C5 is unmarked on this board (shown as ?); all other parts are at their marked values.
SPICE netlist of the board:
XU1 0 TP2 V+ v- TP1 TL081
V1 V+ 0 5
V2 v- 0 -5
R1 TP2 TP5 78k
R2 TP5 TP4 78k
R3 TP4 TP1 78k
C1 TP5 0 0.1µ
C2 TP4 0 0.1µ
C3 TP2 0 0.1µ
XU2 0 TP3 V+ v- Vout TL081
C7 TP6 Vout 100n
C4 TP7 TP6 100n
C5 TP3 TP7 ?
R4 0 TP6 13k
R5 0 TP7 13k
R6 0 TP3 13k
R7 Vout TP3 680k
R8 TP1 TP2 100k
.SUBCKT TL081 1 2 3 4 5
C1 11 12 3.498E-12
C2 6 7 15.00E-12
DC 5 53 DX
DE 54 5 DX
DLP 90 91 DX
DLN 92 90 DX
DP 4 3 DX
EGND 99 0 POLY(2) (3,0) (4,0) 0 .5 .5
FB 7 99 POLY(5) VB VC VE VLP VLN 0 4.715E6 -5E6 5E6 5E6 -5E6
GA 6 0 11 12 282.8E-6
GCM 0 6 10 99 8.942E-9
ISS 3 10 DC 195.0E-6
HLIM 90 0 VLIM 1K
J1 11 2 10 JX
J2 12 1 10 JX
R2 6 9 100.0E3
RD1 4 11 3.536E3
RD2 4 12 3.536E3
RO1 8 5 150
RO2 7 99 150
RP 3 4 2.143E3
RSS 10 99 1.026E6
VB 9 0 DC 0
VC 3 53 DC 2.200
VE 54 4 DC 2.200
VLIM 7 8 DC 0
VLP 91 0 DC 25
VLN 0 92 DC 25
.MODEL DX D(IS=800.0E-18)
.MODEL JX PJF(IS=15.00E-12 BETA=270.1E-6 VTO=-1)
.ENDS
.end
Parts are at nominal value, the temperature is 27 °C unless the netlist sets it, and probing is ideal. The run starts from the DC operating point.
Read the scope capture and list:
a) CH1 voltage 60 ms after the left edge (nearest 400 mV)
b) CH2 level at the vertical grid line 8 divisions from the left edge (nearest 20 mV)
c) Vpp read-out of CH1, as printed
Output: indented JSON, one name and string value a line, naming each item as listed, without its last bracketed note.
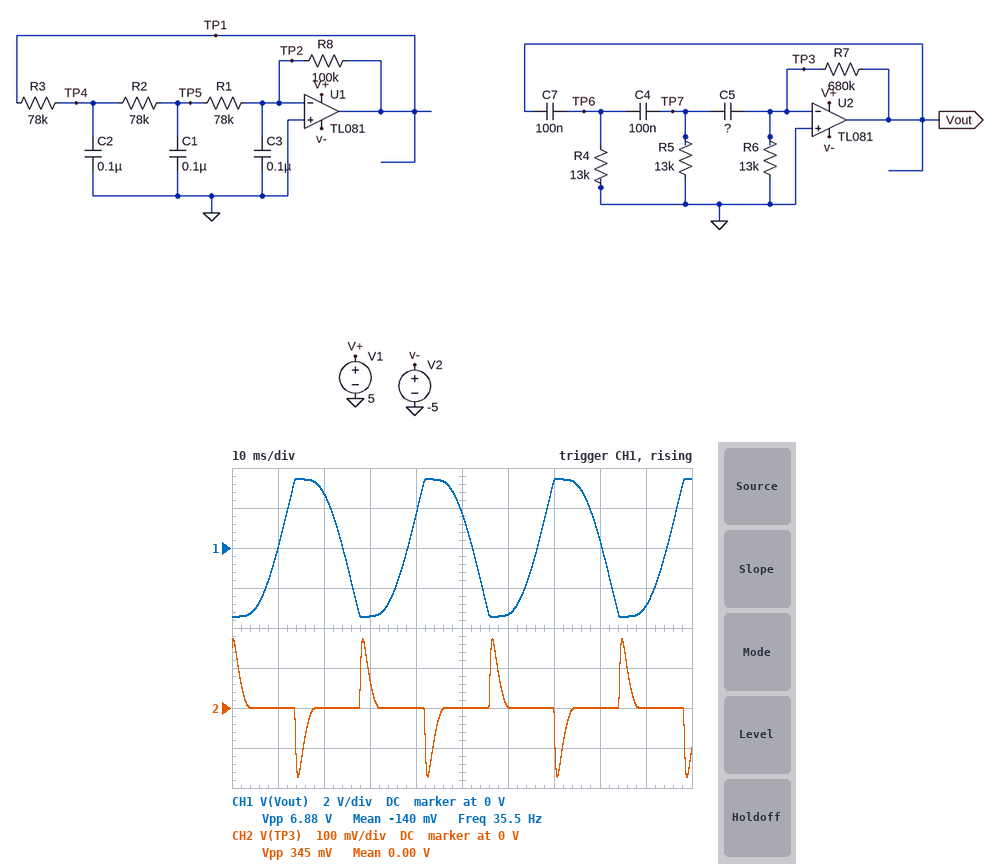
{
  "CH1 voltage 60 ms after the left edge": "-3.2 V",
  "CH2 level at the vertical grid line 8 divisions from the left edge": "0 V",
  "Vpp read-out of CH1, as printed": "6.88 V"
}
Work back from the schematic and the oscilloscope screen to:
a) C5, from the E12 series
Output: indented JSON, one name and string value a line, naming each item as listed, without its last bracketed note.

{
  "C5, from the E12 series": "220 nF"
}
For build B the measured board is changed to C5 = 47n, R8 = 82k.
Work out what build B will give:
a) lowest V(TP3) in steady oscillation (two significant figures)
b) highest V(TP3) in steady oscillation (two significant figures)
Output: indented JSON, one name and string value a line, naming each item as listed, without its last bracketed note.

{
  "lowest V(TP3) in steady oscillation": "-210 mV",
  "highest V(TP3) in steady oscillation": "210 mV"
}
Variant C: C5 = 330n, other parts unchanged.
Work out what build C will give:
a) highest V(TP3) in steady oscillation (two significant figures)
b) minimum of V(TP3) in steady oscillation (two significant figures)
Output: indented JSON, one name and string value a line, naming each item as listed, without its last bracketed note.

{
  "highest V(TP3) in steady oscillation": "140 mV",
  "minimum of V(TP3) in steady oscillation": "-140 mV"
}
